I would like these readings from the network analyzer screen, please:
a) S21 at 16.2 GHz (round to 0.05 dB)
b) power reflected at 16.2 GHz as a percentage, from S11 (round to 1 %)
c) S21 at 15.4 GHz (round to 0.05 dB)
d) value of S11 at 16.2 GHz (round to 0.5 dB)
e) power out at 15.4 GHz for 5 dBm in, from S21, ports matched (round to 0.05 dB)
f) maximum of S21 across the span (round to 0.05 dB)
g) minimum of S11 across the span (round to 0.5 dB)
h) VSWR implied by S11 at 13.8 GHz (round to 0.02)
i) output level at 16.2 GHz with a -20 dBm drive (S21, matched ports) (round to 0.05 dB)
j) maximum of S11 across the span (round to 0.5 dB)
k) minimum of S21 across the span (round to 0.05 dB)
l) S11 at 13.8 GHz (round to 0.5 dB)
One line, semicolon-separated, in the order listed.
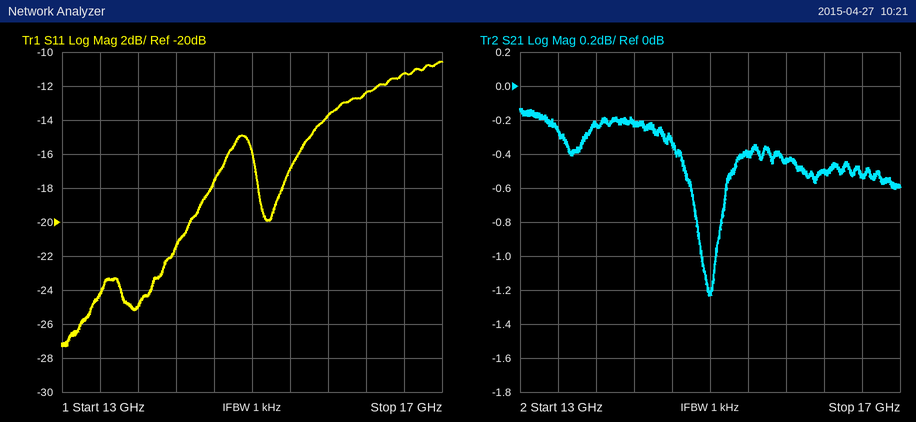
-0.50 dB; 6 %; -0.40 dB; -12.5 dB; 4.60 dBm; -0.15 dB; -27.5 dB; 1.12; -20.50 dBm; -10.5 dB; -1.25 dB; -25.0 dB
